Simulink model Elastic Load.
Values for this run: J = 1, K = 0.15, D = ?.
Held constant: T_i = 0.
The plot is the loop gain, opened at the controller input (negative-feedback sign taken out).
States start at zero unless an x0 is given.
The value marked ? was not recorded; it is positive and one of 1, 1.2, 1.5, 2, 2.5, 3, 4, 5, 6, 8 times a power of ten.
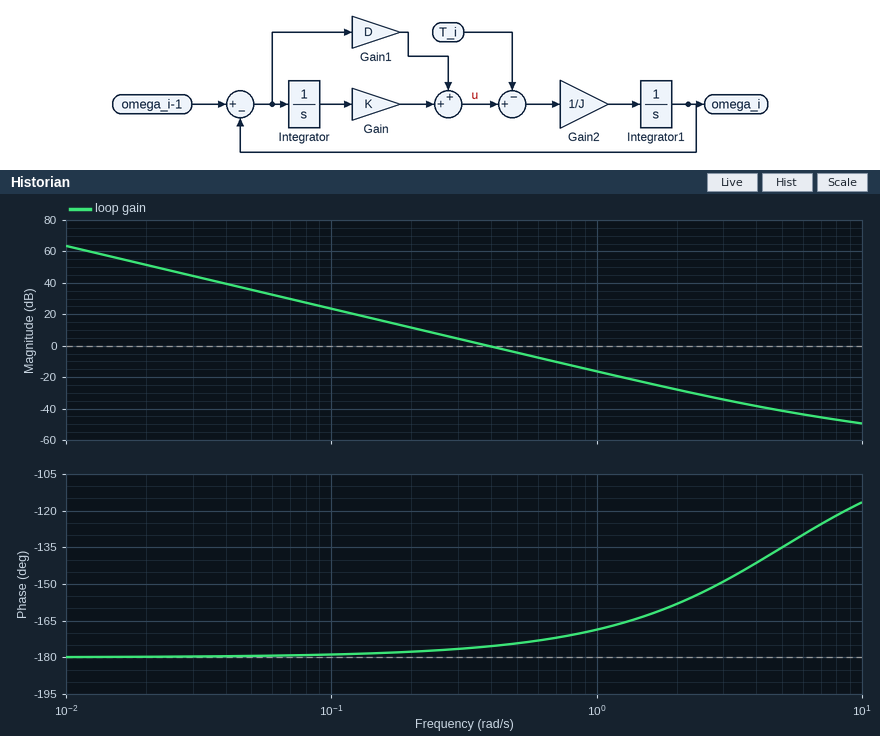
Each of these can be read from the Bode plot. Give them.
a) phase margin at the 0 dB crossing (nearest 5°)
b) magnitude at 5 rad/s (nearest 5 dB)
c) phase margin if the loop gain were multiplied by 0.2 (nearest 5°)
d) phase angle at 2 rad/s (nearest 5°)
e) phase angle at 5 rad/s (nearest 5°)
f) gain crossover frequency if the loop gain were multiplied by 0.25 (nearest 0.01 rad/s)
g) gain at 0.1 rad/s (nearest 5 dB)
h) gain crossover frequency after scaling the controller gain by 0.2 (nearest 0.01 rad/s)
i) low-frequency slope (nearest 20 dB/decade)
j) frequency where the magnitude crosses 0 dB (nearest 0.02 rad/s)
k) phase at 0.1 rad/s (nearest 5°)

5°
-40 dB
0°
-160°
-135°
0.19 rad/s
25 dB
0.17 rad/s
-40 dB/decade
0.38 rad/s
-180°
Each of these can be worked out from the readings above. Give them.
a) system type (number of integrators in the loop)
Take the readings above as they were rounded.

2
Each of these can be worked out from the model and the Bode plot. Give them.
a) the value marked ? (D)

0.03
